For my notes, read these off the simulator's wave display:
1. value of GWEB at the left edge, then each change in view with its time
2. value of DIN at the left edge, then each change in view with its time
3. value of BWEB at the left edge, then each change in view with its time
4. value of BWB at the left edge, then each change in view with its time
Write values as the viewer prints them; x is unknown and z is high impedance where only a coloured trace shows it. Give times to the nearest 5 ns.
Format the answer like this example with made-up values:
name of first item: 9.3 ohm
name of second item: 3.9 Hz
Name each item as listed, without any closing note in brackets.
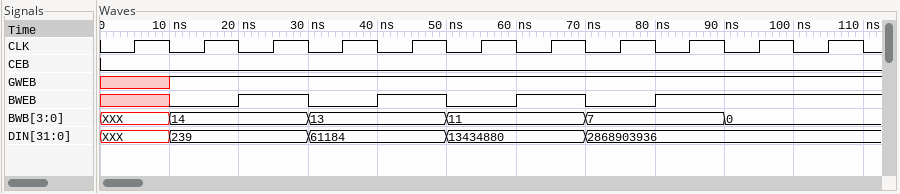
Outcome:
value of GWEB at the left edge, then each change in view with its time: x, 1 at 10 ns
value of DIN at the left edge, then each change in view with its time: XXX, 239 at 10 ns, 61184 at 30 ns, 13434880 at 50 ns, 2868903936 at 70 ns
value of BWEB at the left edge, then each change in view with its time: x, 0 at 10 ns, 1 at 20 ns, 0 at 30 ns, 1 at 40 ns, 0 at 50 ns, 1 at 60 ns, 0 at 70 ns, 1 at 80 ns
value of BWB at the left edge, then each change in view with its time: XXX, 14 at 10 ns, 13 at 30 ns, 11 at 50 ns, 7 at 70 ns, 0 at 90 ns
